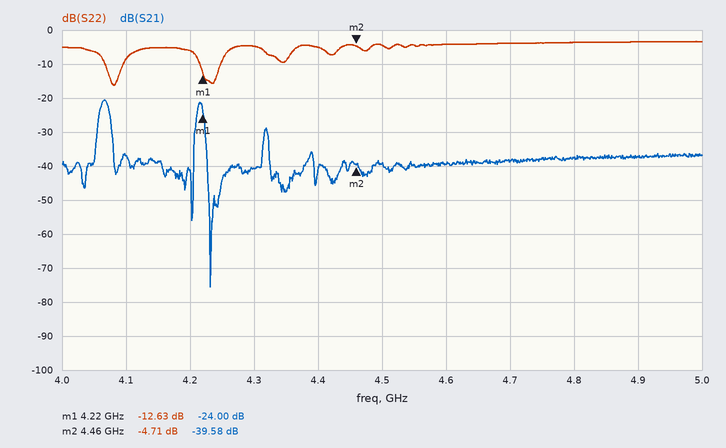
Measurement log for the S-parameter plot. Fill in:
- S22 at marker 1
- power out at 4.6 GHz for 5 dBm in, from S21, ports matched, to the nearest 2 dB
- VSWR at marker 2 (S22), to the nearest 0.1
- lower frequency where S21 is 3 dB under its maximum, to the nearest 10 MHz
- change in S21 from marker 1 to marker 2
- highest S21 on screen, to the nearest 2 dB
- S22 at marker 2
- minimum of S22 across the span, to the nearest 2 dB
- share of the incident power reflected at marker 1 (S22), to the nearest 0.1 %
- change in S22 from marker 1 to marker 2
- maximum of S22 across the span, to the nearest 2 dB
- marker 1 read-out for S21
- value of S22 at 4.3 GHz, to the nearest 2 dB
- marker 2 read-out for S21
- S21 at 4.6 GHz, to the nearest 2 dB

-12.63 dB
-34 dBm
3.8
4.06 GHz
-15.58 dB
-20 dB
-4.71 dB
-16 dB
5.5 %
7.92 dB
-4 dB
-24.00 dB
-4 dB
-39.58 dB
-40 dB
